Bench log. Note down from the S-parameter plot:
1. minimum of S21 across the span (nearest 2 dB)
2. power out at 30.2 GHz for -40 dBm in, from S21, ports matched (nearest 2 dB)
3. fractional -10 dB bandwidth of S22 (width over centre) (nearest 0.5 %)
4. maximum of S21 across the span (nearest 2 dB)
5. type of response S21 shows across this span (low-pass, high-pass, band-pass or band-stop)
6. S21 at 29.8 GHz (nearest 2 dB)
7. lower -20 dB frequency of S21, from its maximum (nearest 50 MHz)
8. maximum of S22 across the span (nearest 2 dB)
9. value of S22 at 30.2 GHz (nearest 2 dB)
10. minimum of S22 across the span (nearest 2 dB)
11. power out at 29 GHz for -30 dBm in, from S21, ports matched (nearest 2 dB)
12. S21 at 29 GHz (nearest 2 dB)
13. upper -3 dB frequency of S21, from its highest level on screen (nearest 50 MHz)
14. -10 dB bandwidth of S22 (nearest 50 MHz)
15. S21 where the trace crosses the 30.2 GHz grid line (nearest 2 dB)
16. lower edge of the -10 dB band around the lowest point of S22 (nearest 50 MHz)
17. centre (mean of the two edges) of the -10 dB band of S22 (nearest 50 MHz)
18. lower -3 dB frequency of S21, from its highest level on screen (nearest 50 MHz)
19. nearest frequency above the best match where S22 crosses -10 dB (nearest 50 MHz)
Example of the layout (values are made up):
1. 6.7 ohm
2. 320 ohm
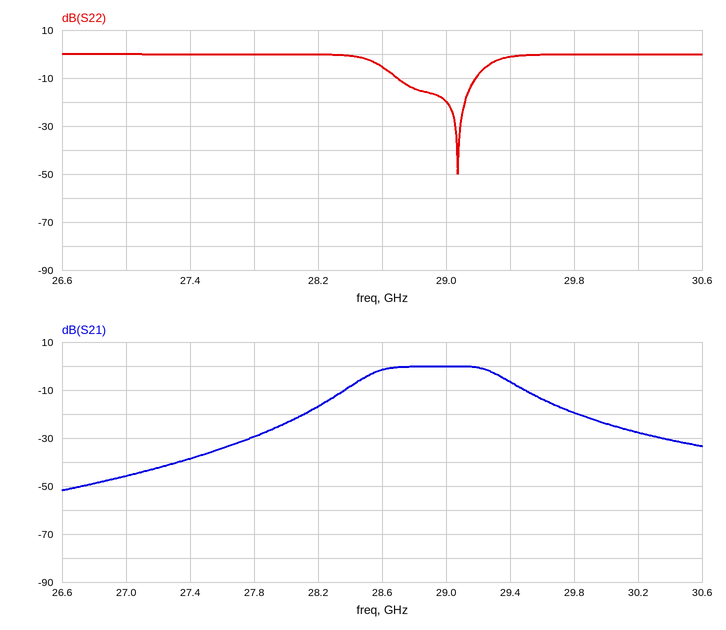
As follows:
1. -52 dB
2. -68 dBm
3. 1.5 %
4. 0 dB
5. band-pass
6. -20 dB
7. 28.10 GHz
8. 0 dB
9. 0 dB
10. -50 dB
11. -30 dBm
12. 0 dB
13. 29.30 GHz
14. 500 MHz
15. -28 dB
16. 28.70 GHz
17. 28.95 GHz
18. 28.55 GHz
19. 29.20 GHz
